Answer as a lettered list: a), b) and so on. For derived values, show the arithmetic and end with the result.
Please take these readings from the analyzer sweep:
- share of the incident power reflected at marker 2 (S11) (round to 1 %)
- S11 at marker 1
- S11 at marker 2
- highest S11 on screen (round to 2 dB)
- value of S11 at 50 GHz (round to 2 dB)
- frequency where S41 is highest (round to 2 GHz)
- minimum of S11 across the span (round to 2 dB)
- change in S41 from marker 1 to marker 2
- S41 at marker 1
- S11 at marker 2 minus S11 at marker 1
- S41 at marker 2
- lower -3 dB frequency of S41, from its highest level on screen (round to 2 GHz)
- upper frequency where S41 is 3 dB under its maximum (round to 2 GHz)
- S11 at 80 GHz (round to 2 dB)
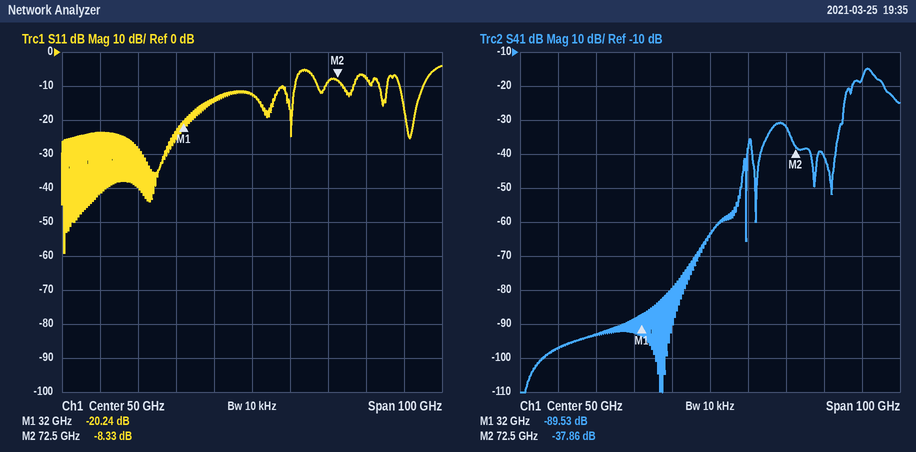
a) 10^(-8.33/10) ≈ 15 %
b) -20.24 dB
c) -8.33 dB
d) -4 dB
e) -12 dB
f) 92 GHz
g) -60 dB
h) -37.86 − (-89.53) = 51.67 dB
i) -89.53 dB
j) -8.33 − (-20.24) = 11.91 dB
k) -37.86 dB
l) 90 GHz
m) 94 GHz
n) -8 dB
